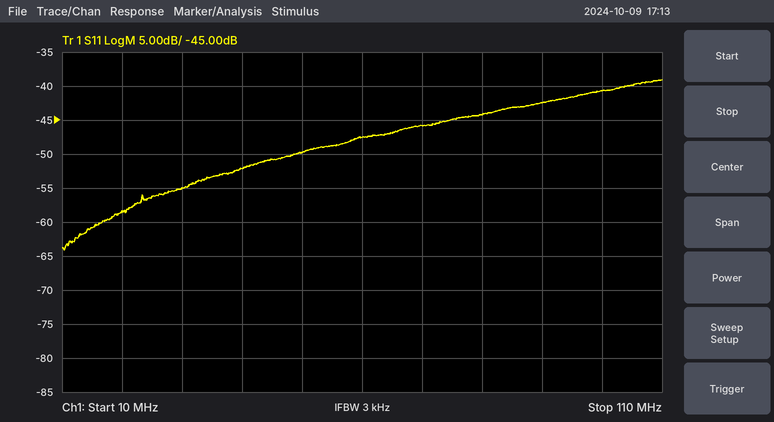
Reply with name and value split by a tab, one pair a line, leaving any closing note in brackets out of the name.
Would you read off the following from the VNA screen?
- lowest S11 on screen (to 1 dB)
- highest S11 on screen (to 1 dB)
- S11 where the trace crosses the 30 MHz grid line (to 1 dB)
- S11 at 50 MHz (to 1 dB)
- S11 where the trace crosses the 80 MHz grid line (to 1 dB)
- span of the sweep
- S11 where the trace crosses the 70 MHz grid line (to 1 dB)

lowest S11 on screen	-64 dB
highest S11 on screen	-39 dB
S11 where the trace crosses the 30 MHz grid line	-55 dB
S11 at 50 MHz	-50 dB
S11 where the trace crosses the 80 MHz grid line	-44 dB
span of the sweep	100 MHz
S11 where the trace crosses the 70 MHz grid line	-46 dB
